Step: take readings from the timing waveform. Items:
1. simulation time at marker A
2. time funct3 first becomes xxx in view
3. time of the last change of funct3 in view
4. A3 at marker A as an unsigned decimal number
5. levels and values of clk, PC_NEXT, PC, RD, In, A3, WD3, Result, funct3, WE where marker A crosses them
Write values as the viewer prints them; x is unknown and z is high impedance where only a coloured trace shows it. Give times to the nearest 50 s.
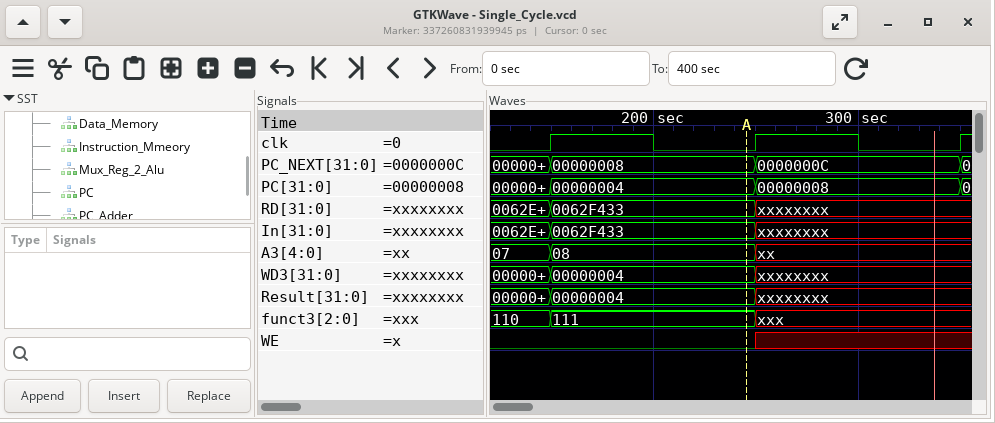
250 s
250 s
250 s
8
clk=0, PC_NEXT=00000008, PC=00000004, RD=0062F433, In=0062F433, A3=08, WD3=00000004, Result=00000004, funct3=111, WE=0
